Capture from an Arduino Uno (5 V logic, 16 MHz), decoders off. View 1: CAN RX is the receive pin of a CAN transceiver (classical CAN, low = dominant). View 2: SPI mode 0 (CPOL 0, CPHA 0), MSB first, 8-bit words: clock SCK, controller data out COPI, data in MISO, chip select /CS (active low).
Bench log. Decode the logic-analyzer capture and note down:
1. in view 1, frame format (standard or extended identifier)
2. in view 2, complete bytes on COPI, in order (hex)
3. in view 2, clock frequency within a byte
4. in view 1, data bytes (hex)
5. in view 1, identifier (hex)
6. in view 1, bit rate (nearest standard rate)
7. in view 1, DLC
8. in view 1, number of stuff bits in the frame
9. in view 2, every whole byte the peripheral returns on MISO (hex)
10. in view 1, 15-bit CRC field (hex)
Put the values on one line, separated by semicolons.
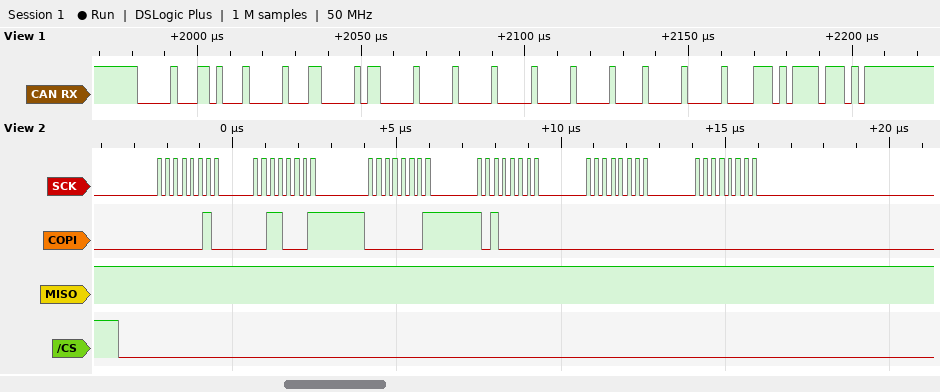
standard; 02 31 01 A0 00 00; 4 MHz; 06 06 00 00 00 00 40 00; 0x00D; 500 kbit/s; 8; 11; FF FF FF FF FF FF; 0x75EE
